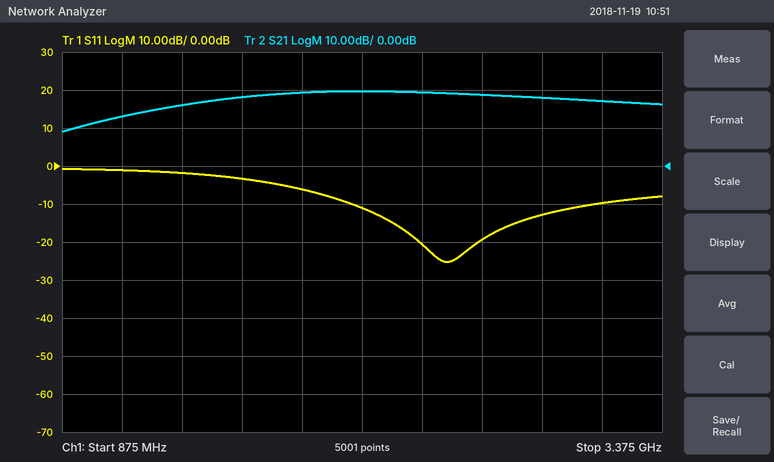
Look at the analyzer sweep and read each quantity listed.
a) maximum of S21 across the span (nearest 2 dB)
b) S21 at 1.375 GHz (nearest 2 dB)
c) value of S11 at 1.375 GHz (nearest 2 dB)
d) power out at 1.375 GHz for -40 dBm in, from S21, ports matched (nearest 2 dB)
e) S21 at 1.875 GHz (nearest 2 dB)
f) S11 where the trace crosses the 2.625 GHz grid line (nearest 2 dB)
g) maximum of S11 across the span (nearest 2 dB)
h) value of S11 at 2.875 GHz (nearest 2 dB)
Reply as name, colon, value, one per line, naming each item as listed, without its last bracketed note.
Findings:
maximum of S21 across the span: 20 dB
S21 at 1.375 GHz: 16 dB
value of S11 at 1.375 GHz: -2 dB
power out at 1.375 GHz for -40 dBm in, from S21, ports matched: -24 dBm
S21 at 1.875 GHz: 20 dB
S11 where the trace crosses the 2.625 GHz grid line: -20 dB
maximum of S11 across the span: 0 dB
value of S11 at 2.875 GHz: -12 dB
